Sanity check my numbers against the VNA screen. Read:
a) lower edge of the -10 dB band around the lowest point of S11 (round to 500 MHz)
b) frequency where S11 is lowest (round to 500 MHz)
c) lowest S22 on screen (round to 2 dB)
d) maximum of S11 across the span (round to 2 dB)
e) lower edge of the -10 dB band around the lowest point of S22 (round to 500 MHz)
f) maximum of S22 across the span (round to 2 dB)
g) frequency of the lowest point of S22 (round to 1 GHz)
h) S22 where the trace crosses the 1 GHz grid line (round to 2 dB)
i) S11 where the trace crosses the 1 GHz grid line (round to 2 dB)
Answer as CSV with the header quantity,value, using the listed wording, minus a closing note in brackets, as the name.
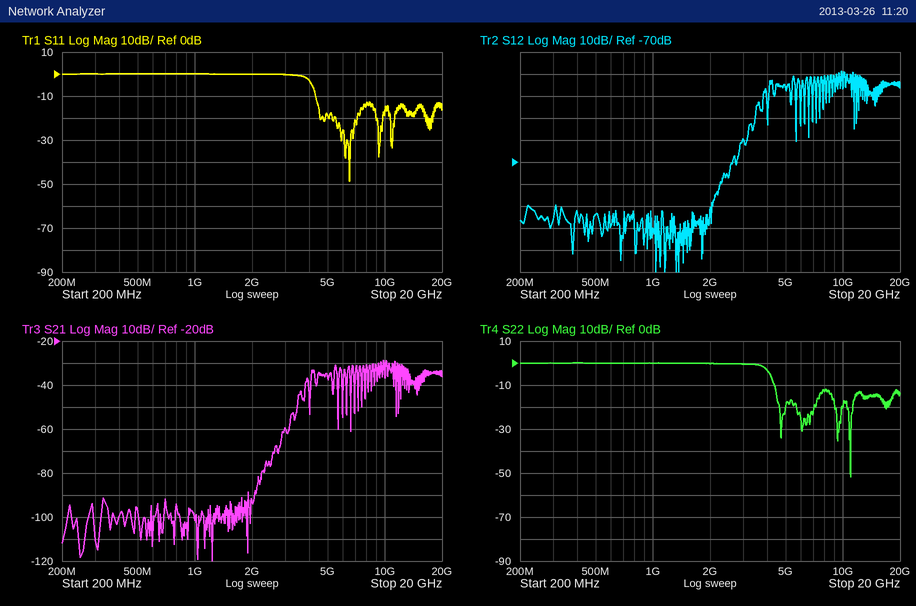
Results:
quantity,value
lower edge of the -10 dB band around the lowest point of S11,4.5 GHz
frequency where S11 is lowest,6.5 GHz
lowest S22 on screen,-52 dB
maximum of S11 across the span,0 dB
lower edge of the -10 dB band around the lowest point of S22,4.5 GHz
maximum of S22 across the span,0 dB
frequency of the lowest point of S22,11 GHz
S22 where the trace crosses the 1 GHz grid line,0 dB
S11 where the trace crosses the 1 GHz grid line,0 dB
